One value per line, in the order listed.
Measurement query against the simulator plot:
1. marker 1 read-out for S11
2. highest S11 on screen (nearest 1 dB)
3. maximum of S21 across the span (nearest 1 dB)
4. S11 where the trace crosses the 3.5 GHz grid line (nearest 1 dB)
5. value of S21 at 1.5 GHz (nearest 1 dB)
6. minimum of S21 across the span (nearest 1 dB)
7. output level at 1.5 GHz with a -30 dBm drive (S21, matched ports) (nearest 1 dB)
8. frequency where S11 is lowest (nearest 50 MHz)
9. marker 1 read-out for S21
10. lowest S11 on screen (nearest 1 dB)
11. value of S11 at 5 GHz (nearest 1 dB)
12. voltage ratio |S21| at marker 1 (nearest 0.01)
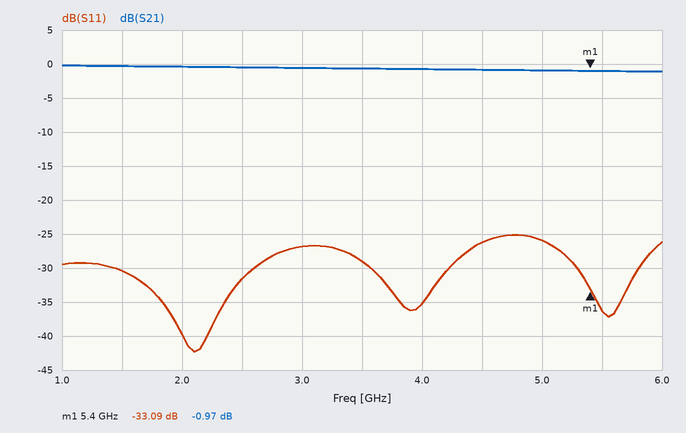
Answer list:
-33.09 dB
-25 dB
0 dB
-29 dB
0 dB
-1 dB
-30 dBm
2.10 GHz
-0.97 dB
-42 dB
-26 dB
0.89
